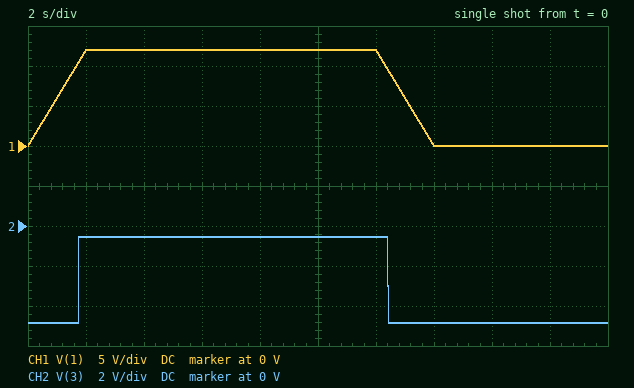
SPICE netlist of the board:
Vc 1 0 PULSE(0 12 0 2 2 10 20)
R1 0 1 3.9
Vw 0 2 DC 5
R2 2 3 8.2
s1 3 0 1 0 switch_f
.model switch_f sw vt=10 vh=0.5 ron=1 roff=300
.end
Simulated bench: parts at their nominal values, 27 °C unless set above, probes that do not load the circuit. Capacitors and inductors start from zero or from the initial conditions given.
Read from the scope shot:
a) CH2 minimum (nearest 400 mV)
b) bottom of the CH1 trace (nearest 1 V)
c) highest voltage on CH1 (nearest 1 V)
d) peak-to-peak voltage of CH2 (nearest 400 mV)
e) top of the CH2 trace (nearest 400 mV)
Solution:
-4.8 V
0 V
12 V
4.4 V
-400 mV
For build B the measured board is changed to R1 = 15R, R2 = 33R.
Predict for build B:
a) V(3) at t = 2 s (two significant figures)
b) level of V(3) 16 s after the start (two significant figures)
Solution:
-150 mV
-4.5 V
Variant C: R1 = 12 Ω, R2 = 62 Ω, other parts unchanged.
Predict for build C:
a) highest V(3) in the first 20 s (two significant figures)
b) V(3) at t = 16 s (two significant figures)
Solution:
-79 mV
-4.1 V
